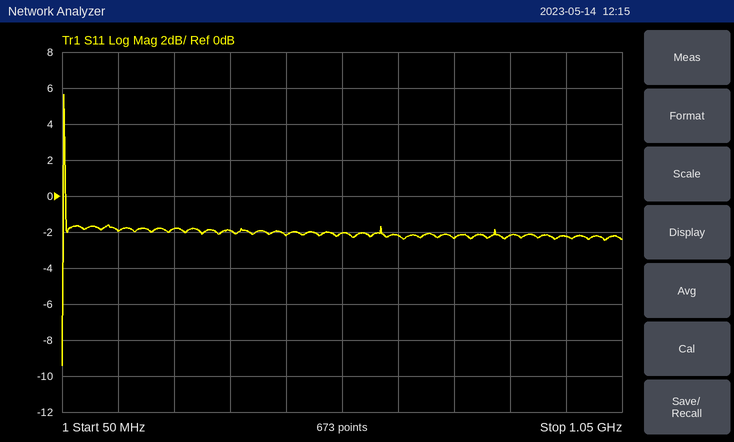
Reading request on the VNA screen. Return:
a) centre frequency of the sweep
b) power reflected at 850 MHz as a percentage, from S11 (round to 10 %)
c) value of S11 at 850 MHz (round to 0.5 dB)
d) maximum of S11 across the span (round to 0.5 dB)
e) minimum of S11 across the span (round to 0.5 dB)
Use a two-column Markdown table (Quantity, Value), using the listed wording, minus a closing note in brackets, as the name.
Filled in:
| Quantity | Value |
|---|---|
| centre frequency of the sweep | 550 MHz |
| power reflected at 850 MHz as a percentage, from S11 | 60 % |
| value of S11 at 850 MHz | -2.0 dB |
| maximum of S11 across the span | 5.5 dB |
| minimum of S11 across the span | -9.5 dB |
